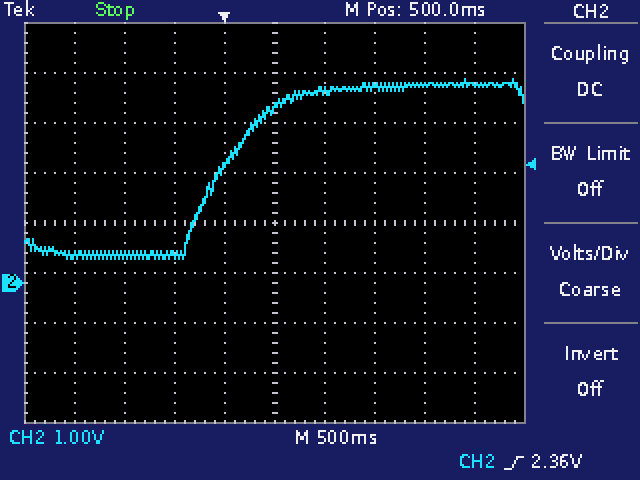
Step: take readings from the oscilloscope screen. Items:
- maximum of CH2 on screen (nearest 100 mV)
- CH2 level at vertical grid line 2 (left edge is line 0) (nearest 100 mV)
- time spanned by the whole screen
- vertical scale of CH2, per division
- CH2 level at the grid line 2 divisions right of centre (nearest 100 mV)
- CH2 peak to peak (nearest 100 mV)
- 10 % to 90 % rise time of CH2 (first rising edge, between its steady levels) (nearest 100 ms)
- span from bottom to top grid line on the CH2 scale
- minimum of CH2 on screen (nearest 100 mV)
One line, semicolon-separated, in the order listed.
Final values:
4.1 V; 600 mV; 5 s; 1 V; 3.9 V; 3.6 V; 900 ms; 8 V; 500 mV
